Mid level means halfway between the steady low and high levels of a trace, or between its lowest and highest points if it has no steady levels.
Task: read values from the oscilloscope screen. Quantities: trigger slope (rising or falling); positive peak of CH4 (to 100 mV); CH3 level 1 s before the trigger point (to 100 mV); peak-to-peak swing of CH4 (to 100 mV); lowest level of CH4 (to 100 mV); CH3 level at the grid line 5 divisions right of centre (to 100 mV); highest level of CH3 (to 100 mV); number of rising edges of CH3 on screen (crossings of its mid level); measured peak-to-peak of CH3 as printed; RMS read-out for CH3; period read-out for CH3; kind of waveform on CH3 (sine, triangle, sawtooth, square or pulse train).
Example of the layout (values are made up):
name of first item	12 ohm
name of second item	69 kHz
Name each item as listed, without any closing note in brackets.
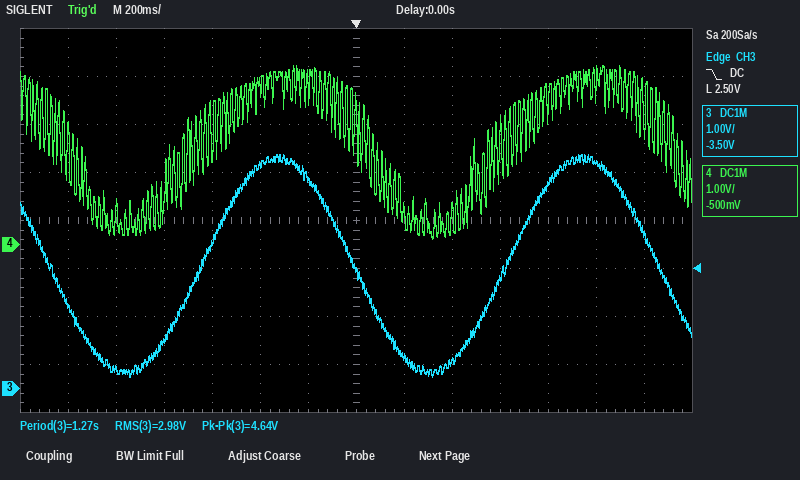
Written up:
trigger slope	falling
positive peak of CH4	3.7 V
CH3 level 1 s before the trigger point	400 mV
peak-to-peak swing of CH4	3.6 V
lowest level of CH4	100 mV
CH3 level at the grid line 5 divisions right of centre	4.7 V
highest level of CH3	4.9 V
number of rising edges of CH3 on screen	2
measured peak-to-peak of CH3 as printed	4.64 V
RMS read-out for CH3	2.98 V
period read-out for CH3	1.27 s
kind of waveform on CH3	sine
